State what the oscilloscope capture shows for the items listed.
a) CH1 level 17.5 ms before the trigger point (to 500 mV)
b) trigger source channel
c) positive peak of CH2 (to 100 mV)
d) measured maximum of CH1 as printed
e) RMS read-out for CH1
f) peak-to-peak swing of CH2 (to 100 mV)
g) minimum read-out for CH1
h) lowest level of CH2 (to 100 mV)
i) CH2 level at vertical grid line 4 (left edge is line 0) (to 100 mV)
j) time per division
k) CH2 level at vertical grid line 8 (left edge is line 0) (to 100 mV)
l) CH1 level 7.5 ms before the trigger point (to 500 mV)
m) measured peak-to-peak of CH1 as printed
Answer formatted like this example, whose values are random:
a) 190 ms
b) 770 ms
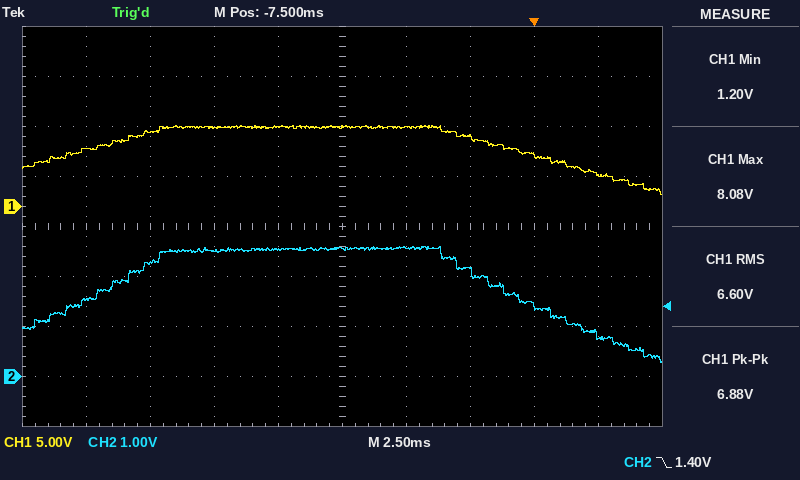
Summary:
a) 6.0 V
b) CH2
c) 2.6 V
d) 8.08 V
e) 6.60 V
f) 2.3 V
g) 1.20 V
h) 300 mV
i) 2.5 V
j) 2.5 ms
k) 1.4 V
l) 8.0 V
m) 6.88 V
